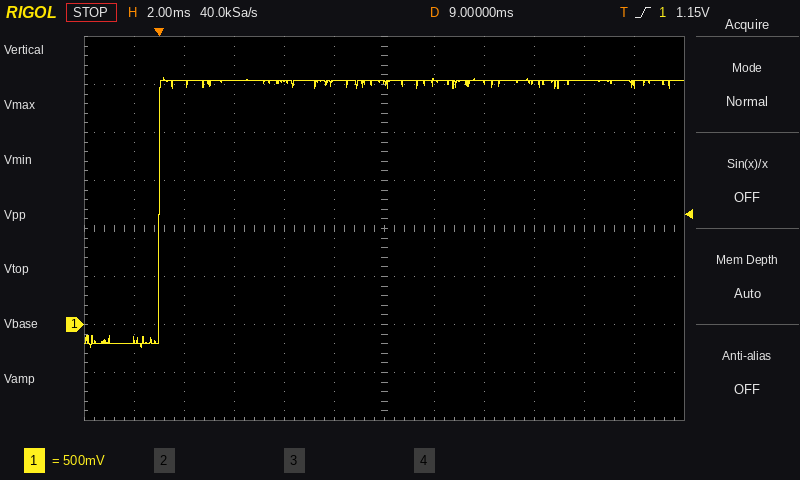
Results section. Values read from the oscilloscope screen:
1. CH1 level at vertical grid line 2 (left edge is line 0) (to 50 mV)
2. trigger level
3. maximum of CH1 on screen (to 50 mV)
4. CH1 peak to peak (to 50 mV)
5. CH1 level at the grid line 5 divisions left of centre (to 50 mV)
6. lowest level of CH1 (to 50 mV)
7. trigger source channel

2.50 V
1.15 V
2.55 V
2.80 V
-150 mV
-250 mV
CH1
